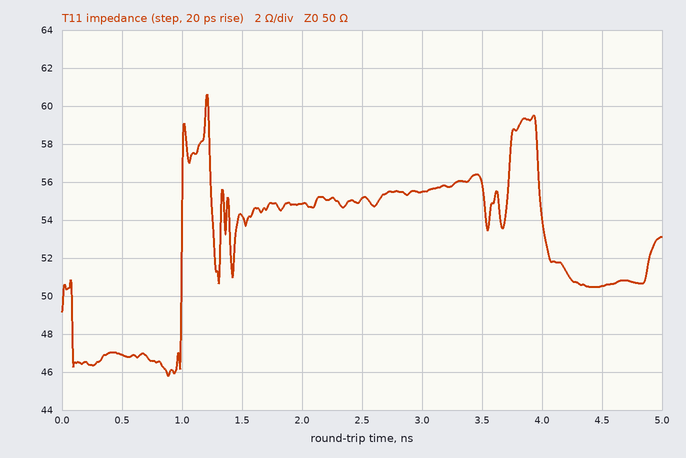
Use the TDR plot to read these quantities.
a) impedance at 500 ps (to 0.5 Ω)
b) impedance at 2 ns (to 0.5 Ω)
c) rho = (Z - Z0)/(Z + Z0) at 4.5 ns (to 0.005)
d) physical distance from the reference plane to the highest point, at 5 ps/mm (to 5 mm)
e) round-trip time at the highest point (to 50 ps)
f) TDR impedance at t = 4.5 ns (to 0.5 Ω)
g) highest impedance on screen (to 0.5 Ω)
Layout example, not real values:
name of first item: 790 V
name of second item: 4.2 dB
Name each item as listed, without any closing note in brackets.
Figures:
impedance at 500 ps: 47.0 Ω
impedance at 2 ns: 55.0 Ω
rho = (Z - Z0)/(Z + Z0) at 4.5 ns: +0.005
physical distance from the reference plane to the highest point, at 5 ps/mm: 120 mm
round-trip time at the highest point: 1.20 ns
TDR impedance at t = 4.5 ns: 50.5 Ω
highest impedance on screen: 60.5 Ω
